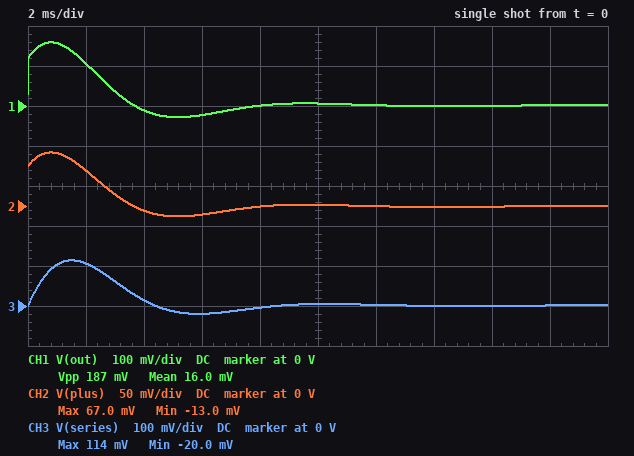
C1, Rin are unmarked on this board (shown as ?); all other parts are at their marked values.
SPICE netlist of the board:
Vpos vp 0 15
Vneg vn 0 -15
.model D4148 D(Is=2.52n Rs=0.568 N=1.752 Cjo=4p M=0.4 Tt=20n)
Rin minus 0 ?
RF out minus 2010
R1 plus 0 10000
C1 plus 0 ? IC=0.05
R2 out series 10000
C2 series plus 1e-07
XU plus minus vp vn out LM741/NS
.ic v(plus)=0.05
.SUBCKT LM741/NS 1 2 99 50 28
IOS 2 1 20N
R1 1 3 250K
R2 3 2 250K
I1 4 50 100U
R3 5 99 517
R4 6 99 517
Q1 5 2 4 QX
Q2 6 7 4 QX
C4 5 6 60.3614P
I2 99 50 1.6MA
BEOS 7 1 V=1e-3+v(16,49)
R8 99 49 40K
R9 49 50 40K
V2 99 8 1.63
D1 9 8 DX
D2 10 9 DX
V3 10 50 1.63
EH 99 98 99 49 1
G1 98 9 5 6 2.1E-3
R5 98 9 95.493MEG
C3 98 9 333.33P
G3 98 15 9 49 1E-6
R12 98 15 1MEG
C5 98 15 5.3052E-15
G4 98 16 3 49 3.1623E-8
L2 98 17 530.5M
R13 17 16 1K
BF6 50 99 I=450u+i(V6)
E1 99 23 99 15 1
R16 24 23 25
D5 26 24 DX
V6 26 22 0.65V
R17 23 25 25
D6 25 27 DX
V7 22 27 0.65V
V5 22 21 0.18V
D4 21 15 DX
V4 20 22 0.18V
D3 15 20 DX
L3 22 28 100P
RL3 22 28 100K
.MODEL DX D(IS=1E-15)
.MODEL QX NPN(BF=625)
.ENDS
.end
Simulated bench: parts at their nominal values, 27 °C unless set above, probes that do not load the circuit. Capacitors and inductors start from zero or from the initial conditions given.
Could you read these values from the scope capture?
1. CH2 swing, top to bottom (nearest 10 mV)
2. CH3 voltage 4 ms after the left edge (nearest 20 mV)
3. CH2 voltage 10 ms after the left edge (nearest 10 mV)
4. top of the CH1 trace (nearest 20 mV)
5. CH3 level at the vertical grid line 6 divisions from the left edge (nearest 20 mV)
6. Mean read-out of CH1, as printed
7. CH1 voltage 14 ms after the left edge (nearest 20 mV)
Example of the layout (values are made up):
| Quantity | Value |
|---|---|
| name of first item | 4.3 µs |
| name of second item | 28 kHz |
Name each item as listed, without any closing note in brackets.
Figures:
| Quantity | Value |
|---|---|
| CH2 swing, top to bottom | 80 mV |
| CH3 voltage 4 ms after the left edge | 20 mV |
| CH2 voltage 10 ms after the left edge | 0 V |
| top of the CH1 trace | 160 mV |
| CH3 level at the vertical grid line 6 divisions from the left edge | 0 V |
| Mean read-out of CH1, as printed | 16.0 mV |
| CH1 voltage 14 ms after the left edge | 0 V |
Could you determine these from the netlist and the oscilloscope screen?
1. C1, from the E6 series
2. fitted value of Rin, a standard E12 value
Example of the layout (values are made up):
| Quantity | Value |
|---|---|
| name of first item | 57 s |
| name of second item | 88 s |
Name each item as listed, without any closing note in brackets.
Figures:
| Quantity | Value |
|---|---|
| C1, from the E6 series | 150 nF |
| fitted value of Rin, a standard E12 value | 1.5 kΩ |
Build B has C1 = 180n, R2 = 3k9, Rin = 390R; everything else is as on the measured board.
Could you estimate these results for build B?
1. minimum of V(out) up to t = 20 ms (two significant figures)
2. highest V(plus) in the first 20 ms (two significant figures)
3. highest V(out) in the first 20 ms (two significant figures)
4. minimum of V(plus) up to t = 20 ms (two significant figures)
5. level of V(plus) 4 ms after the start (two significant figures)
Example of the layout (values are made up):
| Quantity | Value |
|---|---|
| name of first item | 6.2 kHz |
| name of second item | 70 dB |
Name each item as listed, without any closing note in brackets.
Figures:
| Quantity | Value |
|---|---|
| minimum of V(out) up to t = 20 ms | -14 V |
| highest V(plus) in the first 20 ms | 5.9 V |
| highest V(out) in the first 20 ms | 14 V |
| minimum of V(plus) up to t = 20 ms | -5.9 V |
| level of V(plus) 4 ms after the start | -5.6 V |
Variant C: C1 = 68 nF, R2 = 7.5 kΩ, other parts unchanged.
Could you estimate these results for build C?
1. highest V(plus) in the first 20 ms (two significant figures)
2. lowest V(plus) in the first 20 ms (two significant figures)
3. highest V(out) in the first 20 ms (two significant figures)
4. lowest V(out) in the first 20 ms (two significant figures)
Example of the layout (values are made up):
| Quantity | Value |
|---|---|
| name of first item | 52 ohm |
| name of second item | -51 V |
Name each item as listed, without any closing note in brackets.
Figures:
| Quantity | Value |
|---|---|
| highest V(plus) in the first 20 ms | 120 mV |
| lowest V(plus) in the first 20 ms | -98 mV |
| highest V(out) in the first 20 ms | 280 mV |
| lowest V(out) in the first 20 ms | -230 mV |
